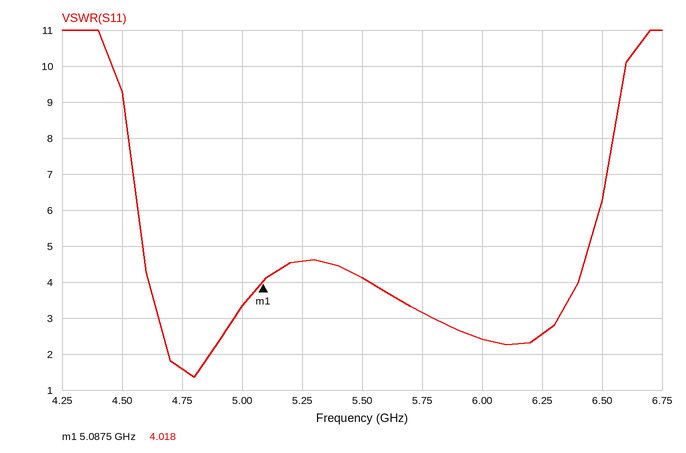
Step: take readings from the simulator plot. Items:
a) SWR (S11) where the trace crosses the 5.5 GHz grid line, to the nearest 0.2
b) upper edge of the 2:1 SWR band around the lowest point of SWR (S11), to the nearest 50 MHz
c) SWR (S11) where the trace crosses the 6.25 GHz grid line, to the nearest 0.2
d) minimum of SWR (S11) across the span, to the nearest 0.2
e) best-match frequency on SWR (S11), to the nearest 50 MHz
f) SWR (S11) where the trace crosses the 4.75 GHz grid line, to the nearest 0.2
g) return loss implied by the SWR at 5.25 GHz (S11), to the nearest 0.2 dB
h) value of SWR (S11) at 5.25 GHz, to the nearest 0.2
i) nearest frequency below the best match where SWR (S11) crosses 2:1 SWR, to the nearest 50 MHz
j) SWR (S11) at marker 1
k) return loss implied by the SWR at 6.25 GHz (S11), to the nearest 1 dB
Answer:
4.2
4.85 GHz
2.6
1.4
4.80 GHz
1.6
3.8 dB
4.6
4.70 GHz
4.018
7 dB
